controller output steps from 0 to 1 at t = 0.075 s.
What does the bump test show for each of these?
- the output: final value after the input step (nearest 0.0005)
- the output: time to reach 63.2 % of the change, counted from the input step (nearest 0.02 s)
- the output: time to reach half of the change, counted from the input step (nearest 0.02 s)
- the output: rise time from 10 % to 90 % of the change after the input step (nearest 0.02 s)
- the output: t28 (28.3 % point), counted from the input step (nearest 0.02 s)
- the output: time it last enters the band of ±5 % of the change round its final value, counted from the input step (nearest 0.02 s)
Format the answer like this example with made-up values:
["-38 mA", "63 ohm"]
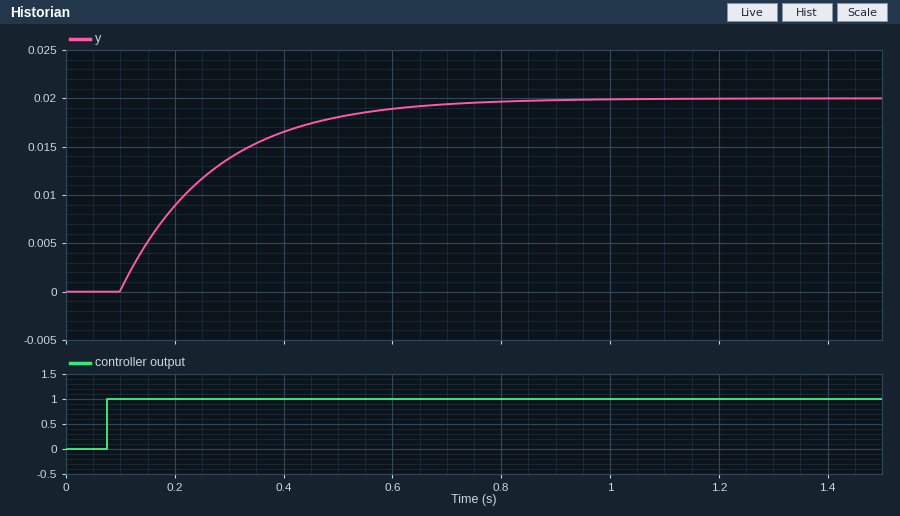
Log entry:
["0.0200", "0.20 s", "0.14 s", "0.38 s", "0.08 s", "0.54 s"]
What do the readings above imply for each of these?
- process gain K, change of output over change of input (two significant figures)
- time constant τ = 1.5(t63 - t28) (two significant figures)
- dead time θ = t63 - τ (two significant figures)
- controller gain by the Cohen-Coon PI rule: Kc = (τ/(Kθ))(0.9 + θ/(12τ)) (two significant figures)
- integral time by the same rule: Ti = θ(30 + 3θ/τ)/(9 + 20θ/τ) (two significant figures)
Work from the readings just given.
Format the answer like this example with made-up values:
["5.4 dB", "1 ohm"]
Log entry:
["0.020", "0.18 s", "0.020 s", "410", "0.054 s"]
